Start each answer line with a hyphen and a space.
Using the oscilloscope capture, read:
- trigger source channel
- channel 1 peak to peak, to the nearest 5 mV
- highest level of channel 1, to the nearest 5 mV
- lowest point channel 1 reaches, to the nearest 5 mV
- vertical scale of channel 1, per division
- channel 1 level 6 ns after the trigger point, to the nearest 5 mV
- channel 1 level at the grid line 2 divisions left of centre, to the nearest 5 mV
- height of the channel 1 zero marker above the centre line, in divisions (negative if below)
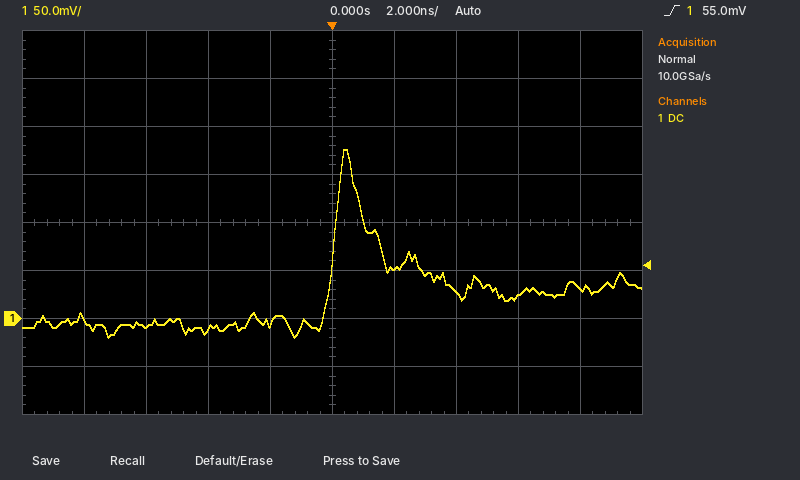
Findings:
- channel 1
- 195 mV
- 175 mV
- -20 mV
- 50 mV
- 25 mV
- -10 mV
- -2.0 div
